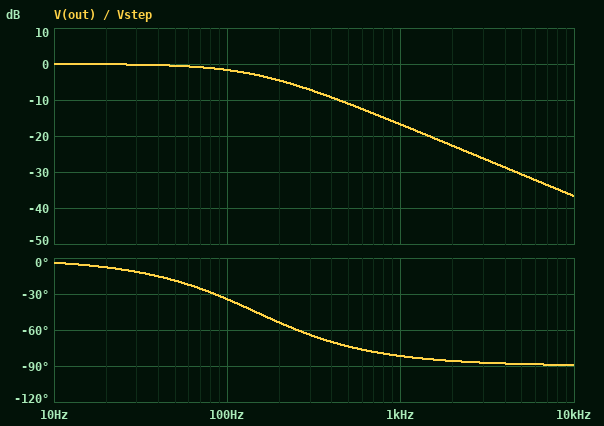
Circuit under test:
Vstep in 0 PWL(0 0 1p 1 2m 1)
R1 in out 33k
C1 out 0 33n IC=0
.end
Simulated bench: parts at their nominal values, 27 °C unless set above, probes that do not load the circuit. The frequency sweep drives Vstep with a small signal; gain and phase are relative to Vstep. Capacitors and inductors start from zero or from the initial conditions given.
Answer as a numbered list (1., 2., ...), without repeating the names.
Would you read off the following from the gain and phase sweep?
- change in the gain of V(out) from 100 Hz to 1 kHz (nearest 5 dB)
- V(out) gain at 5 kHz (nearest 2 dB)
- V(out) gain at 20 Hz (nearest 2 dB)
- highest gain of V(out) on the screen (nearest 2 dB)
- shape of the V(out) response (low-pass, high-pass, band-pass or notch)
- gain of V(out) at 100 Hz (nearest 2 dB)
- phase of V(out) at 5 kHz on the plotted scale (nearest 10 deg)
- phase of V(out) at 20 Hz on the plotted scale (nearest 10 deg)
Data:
1. -15 dB
2. -30 dB
3. 0 dB
4. 0 dB
5. low-pass
6. -2 dB
7. -90 deg
8. -10 deg
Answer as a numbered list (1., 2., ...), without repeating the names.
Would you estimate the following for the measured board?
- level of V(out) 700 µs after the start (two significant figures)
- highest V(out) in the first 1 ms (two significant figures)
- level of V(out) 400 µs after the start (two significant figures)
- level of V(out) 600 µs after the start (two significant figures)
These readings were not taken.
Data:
1. 470 mV
2. 600 mV
3. 310 mV
4. 420 mV
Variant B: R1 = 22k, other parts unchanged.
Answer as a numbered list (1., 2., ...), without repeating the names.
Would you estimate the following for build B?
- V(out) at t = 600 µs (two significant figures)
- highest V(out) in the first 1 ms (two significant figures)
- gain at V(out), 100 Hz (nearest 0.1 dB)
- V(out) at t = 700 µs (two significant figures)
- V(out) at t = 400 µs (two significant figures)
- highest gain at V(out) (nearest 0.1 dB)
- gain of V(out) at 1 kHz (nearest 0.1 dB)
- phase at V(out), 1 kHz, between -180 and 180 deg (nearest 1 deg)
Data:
1. 560 mV
2. 750 mV
3. -0.8 dB
4. 620 mV
5. 420 mV
6. 0 dB
7. -13.4 dB
8. -78 deg
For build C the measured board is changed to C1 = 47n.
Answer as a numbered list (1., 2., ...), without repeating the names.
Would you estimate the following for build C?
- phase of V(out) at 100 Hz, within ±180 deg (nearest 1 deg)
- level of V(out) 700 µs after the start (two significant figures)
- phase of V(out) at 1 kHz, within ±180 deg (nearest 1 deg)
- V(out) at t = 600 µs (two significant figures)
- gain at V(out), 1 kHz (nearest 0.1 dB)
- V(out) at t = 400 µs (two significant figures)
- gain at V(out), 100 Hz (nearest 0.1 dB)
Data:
1. -44 deg
2. 360 mV
3. -84 deg
4. 320 mV
5. -19.8 dB
6. 230 mV
7. -2.9 dB
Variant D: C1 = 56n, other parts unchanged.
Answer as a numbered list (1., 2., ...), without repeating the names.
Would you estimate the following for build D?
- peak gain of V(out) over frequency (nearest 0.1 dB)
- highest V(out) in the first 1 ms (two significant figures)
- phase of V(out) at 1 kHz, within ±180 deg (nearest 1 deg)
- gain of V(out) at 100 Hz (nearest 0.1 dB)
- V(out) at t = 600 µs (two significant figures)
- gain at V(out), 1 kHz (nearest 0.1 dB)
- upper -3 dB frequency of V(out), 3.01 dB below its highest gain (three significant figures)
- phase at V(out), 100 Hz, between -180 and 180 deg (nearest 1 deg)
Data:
1. 0 dB
2. 420 mV
3. -85 deg
4. -3.7 dB
5. 280 mV
6. -21.3 dB
7. 86.1 Hz
8. -49 deg
